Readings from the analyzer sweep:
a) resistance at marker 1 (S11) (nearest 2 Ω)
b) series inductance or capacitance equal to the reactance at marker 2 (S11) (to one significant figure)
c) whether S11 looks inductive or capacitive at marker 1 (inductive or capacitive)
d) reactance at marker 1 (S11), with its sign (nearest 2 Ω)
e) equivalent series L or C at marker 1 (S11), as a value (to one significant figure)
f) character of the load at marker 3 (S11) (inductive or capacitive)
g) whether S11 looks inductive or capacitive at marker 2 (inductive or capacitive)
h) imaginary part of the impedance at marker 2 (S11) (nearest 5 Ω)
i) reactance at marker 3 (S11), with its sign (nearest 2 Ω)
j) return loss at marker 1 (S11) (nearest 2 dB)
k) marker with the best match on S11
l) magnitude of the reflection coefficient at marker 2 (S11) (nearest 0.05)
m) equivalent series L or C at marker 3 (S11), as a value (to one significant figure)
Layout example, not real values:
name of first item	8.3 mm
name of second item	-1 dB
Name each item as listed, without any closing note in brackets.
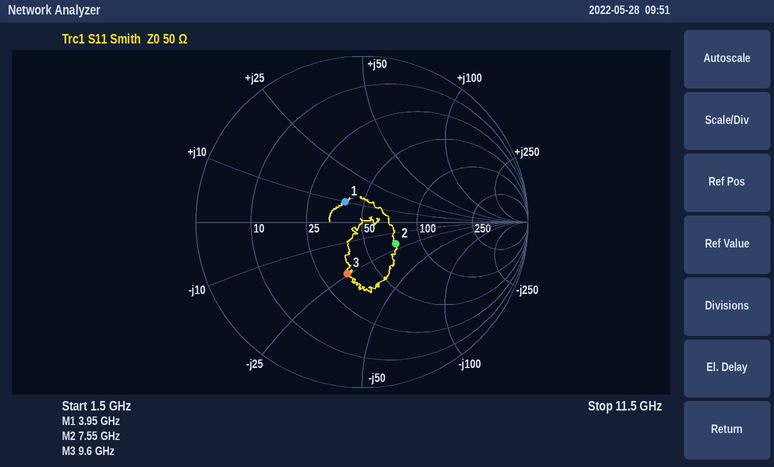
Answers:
resistance at marker 1 (S11)	40 Ω
series inductance or capacitance equal to the reactance at marker 2 (S11)	1 pF
whether S11 looks inductive or capacitive at marker 1	inductive
reactance at marker 1 (S11), with its sign	+10 Ω
equivalent series L or C at marker 1 (S11), as a value	400 pH
character of the load at marker 3 (S11)	capacitive
whether S11 looks inductive or capacitive at marker 2	capacitive
imaginary part of the impedance at marker 2 (S11)	-20 Ω
reactance at marker 3 (S11), with its sign	-24 Ω
return loss at marker 1 (S11)	16 dB
marker with the best match on S11	marker 1
magnitude of the reflection coefficient at marker 2 (S11)	0.25
equivalent series L or C at marker 3 (S11), as a value	700 fF
